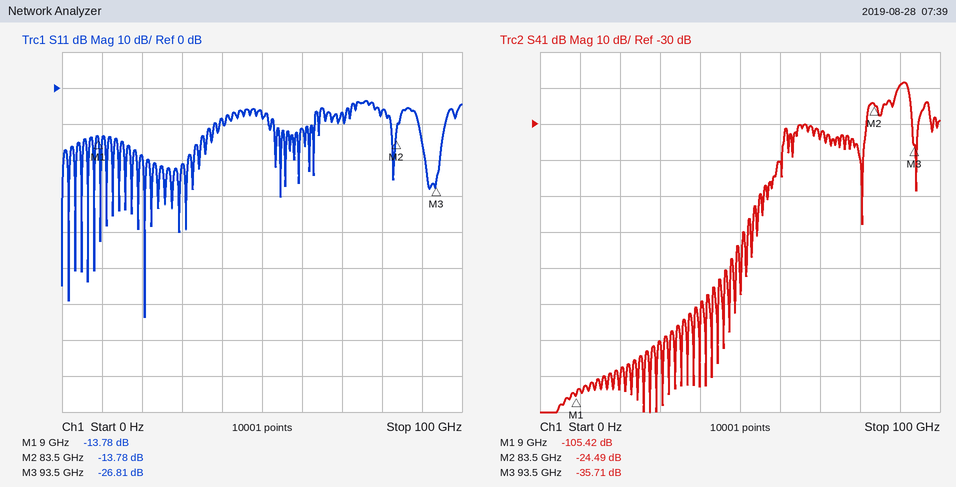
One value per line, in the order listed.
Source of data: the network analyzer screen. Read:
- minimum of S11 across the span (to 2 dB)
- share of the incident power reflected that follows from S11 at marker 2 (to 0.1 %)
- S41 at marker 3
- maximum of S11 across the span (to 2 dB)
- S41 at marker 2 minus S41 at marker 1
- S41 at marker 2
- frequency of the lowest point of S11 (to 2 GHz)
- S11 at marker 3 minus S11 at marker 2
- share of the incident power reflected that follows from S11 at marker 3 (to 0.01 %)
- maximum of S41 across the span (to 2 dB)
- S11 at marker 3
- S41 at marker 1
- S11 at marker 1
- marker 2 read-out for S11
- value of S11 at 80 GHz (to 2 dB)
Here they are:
-64 dB
4.2 %
-35.71 dB
-4 dB
80.93 dB
-24.49 dB
20 GHz
-13.03 dB
0.21 %
-18 dB
-26.81 dB
-105.42 dB
-13.78 dB
-13.78 dB
-6 dB
